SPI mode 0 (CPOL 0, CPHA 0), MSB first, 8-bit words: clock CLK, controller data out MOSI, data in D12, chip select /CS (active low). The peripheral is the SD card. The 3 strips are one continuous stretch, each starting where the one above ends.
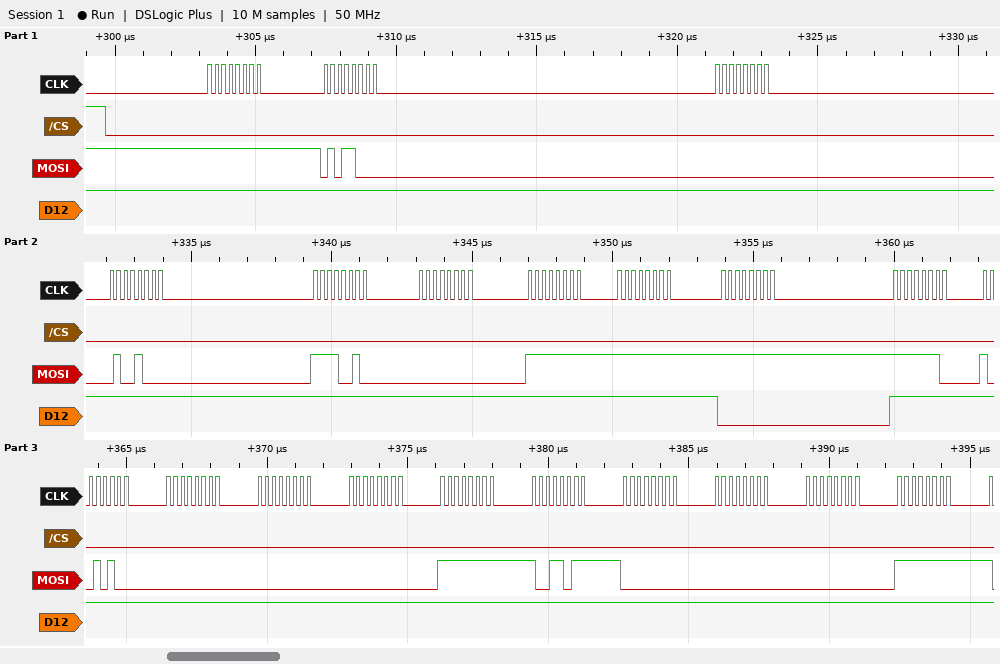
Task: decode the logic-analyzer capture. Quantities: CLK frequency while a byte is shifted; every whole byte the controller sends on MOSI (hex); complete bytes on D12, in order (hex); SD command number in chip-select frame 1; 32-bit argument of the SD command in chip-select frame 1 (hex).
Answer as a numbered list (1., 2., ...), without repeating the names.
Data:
1. 4 MHz
2. FF 58 00 48 F2 00 FF FF FF FE 94 00 00 00 FF 9B 00 00 00 FF
3. FF FF FF FF FF FF FF FF 00 FF FF FF FF FF FF FF FF FF FF FF
4. CMD24
5. 0x0048F200
